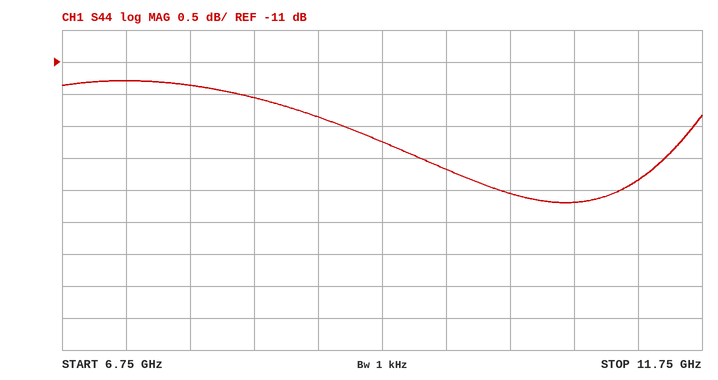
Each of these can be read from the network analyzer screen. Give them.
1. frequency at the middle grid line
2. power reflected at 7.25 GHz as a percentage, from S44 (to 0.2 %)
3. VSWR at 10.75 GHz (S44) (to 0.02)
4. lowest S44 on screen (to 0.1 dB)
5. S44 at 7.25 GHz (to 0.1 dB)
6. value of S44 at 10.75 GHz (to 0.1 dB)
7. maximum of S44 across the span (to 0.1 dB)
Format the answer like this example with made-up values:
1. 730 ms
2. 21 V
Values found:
1. 9.25 GHz
2. 7.4 %
3. 1.56
4. -13.2 dB
5. -11.3 dB
6. -13.2 dB
7. -11.3 dB
